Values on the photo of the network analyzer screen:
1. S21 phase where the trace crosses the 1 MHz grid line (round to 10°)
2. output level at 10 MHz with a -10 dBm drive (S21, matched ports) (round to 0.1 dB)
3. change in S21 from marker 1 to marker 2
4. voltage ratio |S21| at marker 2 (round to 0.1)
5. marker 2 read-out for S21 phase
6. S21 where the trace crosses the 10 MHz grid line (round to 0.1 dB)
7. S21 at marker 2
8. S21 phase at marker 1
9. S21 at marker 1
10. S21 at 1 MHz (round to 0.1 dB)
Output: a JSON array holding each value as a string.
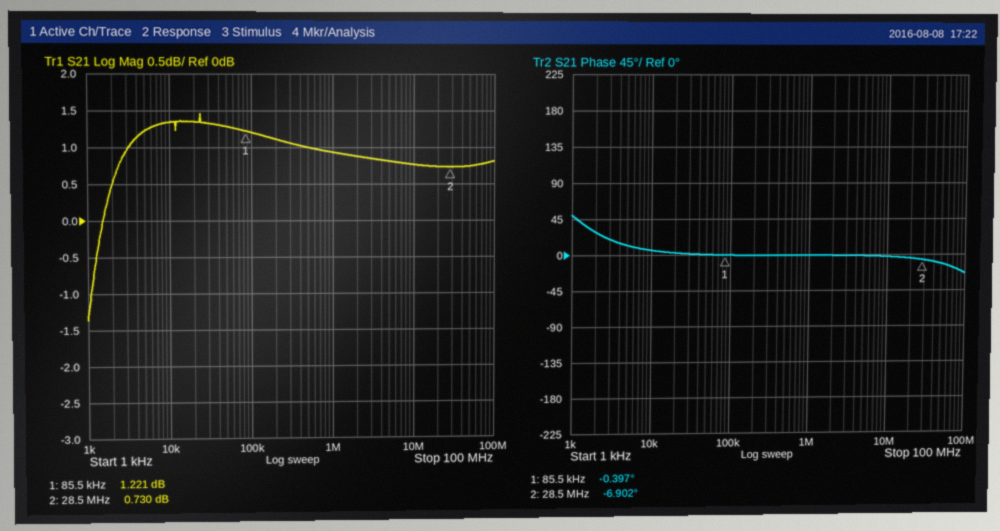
["0°", "-9.2 dBm", "-0.491 dB", "1.1", "-6.902°", "0.8 dB", "0.730 dB", "-0.397°", "1.221 dB", "0.9 dB"]
